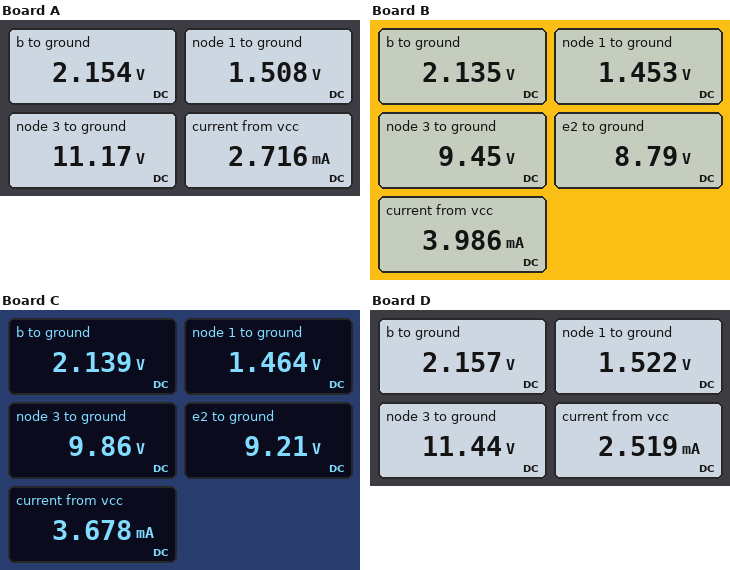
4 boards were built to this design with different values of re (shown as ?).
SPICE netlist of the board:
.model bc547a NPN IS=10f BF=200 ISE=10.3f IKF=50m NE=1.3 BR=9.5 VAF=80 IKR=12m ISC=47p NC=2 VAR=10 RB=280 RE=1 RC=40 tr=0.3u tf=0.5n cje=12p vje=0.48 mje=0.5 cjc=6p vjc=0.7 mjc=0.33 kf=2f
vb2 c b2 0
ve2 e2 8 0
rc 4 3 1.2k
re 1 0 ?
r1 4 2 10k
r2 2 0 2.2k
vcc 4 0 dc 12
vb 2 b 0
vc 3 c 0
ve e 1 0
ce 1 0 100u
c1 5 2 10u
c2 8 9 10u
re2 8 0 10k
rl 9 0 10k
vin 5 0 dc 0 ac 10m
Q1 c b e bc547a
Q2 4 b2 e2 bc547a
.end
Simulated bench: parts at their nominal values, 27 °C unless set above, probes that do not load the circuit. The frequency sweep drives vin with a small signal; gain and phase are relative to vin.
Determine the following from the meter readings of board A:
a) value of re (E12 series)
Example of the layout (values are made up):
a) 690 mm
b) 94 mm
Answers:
a) 2.2 kΩ
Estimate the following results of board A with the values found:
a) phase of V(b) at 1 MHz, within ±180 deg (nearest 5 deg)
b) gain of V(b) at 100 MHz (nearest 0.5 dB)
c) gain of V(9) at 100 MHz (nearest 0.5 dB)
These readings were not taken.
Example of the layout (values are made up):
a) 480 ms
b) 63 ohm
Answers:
a) 0 deg
b) 0 dB
c) -7.5 dB
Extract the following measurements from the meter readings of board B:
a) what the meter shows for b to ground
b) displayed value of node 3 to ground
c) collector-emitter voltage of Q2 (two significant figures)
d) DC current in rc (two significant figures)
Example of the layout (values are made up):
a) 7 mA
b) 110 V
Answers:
a) 2.135 V
b) 9.45 V
c) 3.2 V
d) 2.1 mA
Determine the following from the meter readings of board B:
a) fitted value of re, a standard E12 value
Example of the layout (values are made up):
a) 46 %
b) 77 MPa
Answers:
a) 680 Ω
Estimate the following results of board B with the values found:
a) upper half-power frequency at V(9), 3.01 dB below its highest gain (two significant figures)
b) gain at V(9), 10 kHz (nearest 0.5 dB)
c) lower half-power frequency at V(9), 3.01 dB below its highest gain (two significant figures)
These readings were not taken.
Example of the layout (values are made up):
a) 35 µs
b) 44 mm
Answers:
a) 2.0 MHz
b) 37.5 dB
c) 110 Hz
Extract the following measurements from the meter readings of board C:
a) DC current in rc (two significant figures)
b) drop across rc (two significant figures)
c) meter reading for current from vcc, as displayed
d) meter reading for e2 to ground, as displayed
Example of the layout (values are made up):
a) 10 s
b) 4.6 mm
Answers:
a) 1.8 mA
b) 2.1 V
c) 3.678 mA
d) 9.21 V
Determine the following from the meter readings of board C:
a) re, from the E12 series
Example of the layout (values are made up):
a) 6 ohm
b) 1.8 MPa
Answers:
a) 820 Ω
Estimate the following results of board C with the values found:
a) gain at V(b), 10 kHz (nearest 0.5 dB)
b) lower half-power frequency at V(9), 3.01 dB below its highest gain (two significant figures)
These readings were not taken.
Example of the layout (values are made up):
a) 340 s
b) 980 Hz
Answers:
a) 0 dB
b) 96 Hz
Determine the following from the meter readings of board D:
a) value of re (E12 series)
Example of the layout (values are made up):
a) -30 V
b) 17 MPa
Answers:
a) 3.3 kΩ
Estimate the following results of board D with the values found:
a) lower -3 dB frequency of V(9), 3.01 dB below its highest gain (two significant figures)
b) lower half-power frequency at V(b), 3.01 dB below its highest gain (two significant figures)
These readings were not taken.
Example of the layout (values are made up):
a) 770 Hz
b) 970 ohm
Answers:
a) 32 Hz
b) 9.8 Hz
